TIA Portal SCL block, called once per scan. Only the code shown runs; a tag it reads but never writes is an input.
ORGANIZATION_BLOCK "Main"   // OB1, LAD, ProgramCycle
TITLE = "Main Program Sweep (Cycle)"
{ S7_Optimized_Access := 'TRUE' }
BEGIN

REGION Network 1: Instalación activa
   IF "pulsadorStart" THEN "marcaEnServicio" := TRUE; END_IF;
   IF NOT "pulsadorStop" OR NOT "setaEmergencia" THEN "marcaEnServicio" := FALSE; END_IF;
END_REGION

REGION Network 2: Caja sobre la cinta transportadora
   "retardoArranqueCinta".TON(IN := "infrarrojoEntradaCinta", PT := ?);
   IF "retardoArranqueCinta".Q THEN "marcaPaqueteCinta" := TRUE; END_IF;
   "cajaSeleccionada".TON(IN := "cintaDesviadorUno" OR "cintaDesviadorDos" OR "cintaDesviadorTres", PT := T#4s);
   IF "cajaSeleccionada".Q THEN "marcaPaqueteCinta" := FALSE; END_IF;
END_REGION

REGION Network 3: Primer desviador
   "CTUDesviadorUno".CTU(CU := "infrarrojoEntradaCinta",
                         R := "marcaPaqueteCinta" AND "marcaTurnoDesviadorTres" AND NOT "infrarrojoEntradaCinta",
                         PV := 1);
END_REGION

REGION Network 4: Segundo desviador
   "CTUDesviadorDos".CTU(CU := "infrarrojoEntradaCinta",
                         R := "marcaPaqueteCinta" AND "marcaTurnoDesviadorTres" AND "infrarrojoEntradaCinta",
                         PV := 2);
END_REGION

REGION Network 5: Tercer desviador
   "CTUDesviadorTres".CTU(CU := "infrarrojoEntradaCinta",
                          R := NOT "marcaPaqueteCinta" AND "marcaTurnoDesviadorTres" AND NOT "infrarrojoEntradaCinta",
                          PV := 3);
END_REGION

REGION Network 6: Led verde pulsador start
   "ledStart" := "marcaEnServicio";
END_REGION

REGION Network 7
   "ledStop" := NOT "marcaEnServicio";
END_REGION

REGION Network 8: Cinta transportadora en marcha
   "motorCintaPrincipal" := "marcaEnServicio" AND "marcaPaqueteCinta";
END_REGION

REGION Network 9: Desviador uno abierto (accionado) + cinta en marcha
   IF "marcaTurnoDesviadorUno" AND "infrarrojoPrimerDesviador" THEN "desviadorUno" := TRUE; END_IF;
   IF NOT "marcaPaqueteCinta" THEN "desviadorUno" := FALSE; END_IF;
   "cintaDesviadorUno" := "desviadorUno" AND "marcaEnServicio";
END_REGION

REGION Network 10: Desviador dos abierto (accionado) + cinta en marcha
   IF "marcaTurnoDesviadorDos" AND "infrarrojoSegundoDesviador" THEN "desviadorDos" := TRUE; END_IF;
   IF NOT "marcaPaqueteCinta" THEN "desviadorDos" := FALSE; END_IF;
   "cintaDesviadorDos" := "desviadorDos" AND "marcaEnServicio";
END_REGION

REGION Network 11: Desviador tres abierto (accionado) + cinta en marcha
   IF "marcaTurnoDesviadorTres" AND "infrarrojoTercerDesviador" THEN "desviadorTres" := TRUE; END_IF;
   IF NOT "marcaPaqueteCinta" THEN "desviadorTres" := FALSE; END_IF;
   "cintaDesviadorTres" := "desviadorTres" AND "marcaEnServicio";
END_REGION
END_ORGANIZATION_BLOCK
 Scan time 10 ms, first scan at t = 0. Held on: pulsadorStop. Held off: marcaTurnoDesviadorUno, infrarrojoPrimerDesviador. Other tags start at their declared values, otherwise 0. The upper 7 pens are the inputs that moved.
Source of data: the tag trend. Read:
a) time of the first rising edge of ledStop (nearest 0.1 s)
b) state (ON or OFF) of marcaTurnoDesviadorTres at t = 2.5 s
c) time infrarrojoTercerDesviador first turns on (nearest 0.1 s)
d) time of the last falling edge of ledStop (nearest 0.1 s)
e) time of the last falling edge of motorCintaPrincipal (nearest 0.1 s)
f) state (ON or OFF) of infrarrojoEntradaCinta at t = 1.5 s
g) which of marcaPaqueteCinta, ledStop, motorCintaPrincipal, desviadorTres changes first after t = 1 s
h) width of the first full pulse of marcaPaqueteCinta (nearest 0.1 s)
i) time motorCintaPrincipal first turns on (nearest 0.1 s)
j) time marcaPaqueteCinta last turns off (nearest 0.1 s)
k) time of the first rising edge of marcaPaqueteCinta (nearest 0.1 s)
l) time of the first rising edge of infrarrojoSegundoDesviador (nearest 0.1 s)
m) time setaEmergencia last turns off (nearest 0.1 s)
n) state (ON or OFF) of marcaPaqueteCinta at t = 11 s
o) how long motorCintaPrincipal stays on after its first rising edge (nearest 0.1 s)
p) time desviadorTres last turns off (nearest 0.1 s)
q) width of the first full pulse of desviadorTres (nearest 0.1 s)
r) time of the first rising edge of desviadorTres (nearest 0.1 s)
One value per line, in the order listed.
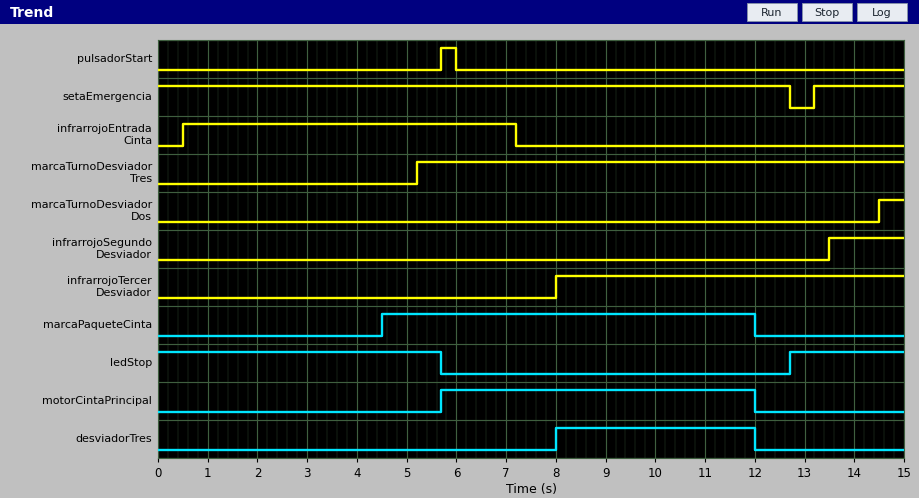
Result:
12.7 s
OFF
8.0 s
5.7 s
12.0 s
ON
marcaPaqueteCinta
7.5 s
5.7 s
12.0 s
4.5 s
13.5 s
12.7 s
ON
6.3 s
12.0 s
4.0 s
8.0 s
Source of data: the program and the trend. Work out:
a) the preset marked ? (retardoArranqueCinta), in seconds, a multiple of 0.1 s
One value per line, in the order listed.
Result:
4.0 s
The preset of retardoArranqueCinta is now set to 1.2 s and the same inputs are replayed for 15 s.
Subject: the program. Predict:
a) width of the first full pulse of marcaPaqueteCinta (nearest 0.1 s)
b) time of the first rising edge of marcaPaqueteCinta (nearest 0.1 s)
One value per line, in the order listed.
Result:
10.3 s
1.7 s
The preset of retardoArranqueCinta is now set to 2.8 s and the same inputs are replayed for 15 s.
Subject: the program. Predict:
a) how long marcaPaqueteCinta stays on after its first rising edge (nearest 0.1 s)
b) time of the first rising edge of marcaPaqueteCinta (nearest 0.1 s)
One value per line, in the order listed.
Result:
8.7 s
3.3 s
